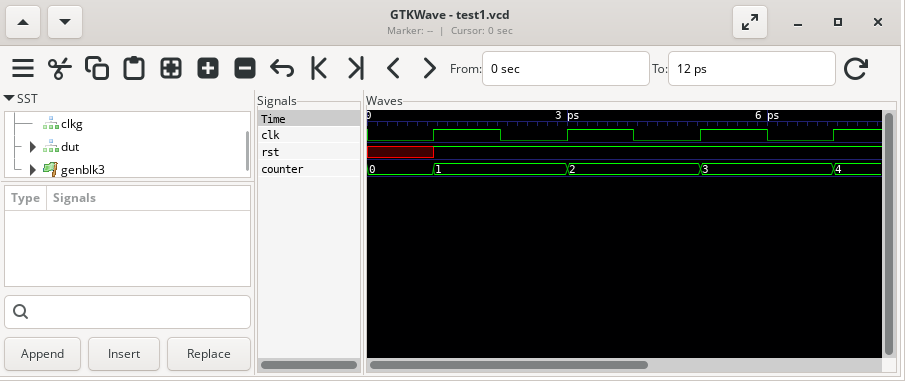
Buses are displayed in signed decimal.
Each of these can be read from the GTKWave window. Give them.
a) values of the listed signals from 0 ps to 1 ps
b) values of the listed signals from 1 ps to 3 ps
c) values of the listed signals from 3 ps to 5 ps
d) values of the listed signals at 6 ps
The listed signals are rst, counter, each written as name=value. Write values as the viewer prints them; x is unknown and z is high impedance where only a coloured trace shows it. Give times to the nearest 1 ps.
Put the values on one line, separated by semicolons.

rst=x, counter=0; rst=1, counter=1; rst=1, counter=2; rst=1, counter=3
